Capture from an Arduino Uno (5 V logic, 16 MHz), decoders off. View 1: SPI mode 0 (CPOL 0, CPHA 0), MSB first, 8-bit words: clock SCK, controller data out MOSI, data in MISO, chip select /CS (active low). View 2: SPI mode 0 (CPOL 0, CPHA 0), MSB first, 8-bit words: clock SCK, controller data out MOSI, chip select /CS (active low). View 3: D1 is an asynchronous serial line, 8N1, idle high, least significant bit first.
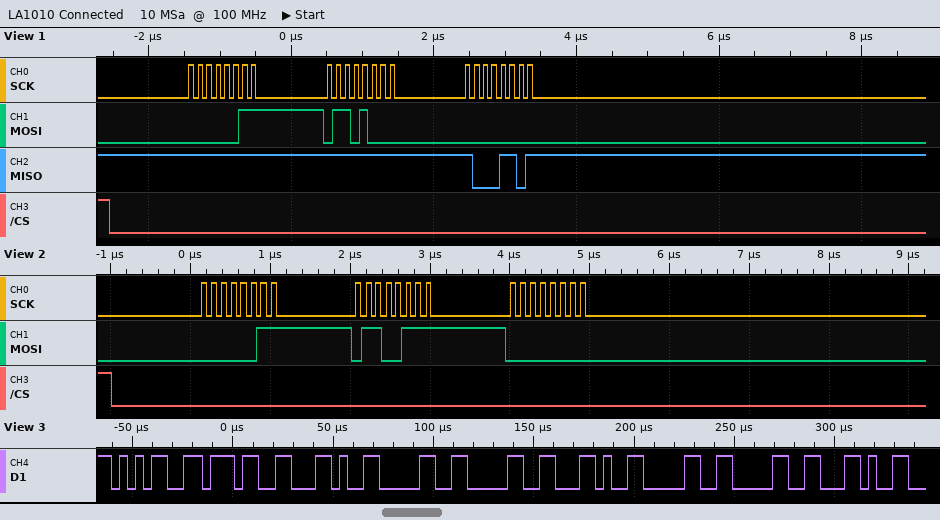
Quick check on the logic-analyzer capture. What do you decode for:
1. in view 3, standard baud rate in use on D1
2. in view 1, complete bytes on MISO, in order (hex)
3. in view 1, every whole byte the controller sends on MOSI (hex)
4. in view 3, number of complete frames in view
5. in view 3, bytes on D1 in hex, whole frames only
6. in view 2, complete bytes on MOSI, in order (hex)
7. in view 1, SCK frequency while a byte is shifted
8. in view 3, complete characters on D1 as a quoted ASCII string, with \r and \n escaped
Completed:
250000 baud
FF FF 8D
03 68 00
9
0x35 0x37 0x2C 0x30 0x30 0x2C 0x30 0x30 0x2C
0x03 0x67 0x00
8 MHz
"57,00,00,"
